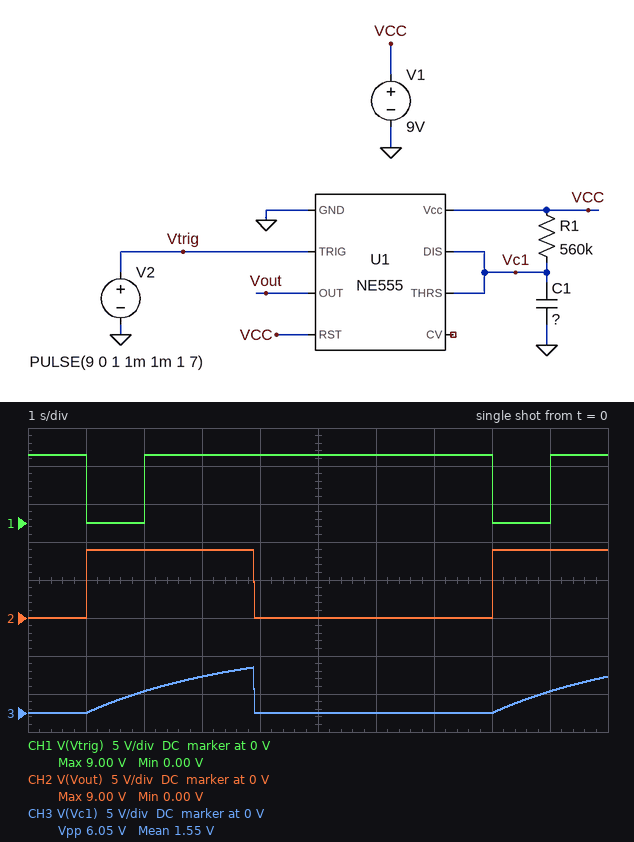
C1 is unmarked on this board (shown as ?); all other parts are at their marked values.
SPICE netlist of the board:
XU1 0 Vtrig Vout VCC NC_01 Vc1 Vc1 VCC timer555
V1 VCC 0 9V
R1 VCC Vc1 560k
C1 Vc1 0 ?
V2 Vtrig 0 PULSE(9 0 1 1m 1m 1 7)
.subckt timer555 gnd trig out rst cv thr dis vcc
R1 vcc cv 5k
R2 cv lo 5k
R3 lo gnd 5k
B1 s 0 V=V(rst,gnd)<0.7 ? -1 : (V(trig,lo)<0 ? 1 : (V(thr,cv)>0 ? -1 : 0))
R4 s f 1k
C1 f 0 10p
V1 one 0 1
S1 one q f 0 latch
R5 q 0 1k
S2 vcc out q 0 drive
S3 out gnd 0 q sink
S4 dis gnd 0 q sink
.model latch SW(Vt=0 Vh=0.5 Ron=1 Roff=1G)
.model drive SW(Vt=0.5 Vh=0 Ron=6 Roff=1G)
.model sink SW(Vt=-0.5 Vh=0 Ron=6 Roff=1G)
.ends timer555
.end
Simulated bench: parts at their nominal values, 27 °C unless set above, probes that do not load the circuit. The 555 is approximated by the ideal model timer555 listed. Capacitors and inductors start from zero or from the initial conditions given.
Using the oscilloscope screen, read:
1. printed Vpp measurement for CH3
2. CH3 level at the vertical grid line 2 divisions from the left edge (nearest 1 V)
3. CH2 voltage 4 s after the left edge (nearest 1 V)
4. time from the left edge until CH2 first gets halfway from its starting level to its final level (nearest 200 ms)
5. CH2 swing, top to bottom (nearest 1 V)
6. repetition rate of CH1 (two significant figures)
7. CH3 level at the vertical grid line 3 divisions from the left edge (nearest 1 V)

6.05 V
3 V
0 V
1.0 s
9 V
140 mHz
5 V
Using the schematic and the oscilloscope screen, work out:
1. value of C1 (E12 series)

4.7 µF
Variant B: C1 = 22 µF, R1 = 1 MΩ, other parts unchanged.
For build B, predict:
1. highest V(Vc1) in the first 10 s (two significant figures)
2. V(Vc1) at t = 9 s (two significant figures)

3.0 V
2.7 V
